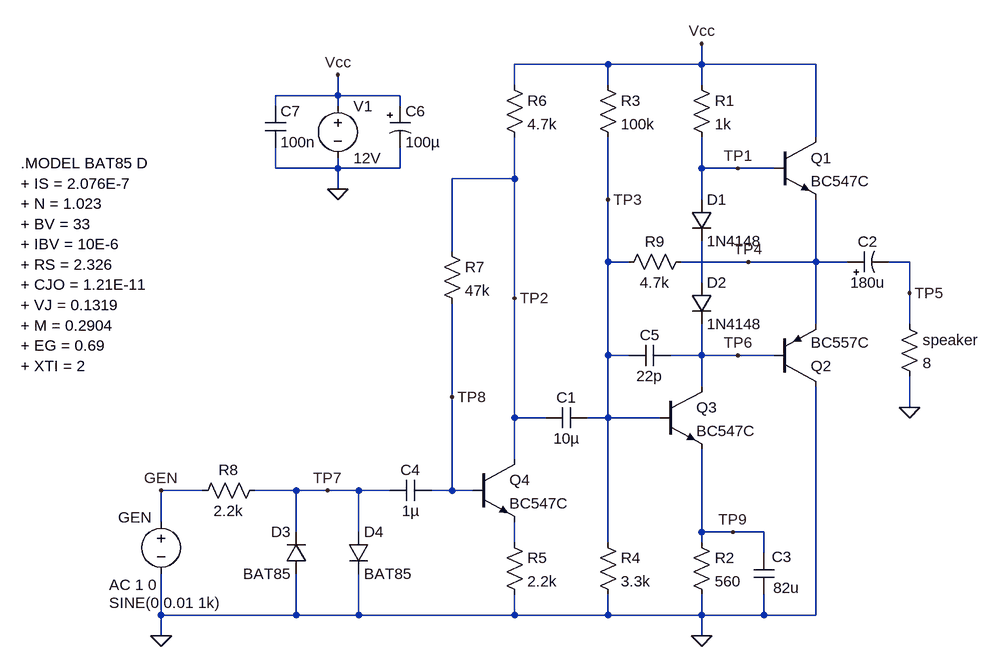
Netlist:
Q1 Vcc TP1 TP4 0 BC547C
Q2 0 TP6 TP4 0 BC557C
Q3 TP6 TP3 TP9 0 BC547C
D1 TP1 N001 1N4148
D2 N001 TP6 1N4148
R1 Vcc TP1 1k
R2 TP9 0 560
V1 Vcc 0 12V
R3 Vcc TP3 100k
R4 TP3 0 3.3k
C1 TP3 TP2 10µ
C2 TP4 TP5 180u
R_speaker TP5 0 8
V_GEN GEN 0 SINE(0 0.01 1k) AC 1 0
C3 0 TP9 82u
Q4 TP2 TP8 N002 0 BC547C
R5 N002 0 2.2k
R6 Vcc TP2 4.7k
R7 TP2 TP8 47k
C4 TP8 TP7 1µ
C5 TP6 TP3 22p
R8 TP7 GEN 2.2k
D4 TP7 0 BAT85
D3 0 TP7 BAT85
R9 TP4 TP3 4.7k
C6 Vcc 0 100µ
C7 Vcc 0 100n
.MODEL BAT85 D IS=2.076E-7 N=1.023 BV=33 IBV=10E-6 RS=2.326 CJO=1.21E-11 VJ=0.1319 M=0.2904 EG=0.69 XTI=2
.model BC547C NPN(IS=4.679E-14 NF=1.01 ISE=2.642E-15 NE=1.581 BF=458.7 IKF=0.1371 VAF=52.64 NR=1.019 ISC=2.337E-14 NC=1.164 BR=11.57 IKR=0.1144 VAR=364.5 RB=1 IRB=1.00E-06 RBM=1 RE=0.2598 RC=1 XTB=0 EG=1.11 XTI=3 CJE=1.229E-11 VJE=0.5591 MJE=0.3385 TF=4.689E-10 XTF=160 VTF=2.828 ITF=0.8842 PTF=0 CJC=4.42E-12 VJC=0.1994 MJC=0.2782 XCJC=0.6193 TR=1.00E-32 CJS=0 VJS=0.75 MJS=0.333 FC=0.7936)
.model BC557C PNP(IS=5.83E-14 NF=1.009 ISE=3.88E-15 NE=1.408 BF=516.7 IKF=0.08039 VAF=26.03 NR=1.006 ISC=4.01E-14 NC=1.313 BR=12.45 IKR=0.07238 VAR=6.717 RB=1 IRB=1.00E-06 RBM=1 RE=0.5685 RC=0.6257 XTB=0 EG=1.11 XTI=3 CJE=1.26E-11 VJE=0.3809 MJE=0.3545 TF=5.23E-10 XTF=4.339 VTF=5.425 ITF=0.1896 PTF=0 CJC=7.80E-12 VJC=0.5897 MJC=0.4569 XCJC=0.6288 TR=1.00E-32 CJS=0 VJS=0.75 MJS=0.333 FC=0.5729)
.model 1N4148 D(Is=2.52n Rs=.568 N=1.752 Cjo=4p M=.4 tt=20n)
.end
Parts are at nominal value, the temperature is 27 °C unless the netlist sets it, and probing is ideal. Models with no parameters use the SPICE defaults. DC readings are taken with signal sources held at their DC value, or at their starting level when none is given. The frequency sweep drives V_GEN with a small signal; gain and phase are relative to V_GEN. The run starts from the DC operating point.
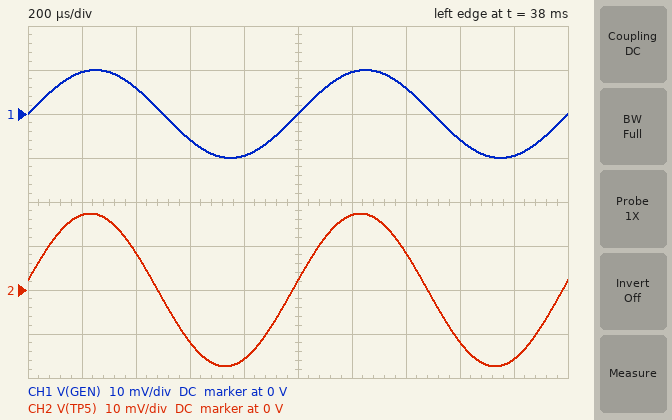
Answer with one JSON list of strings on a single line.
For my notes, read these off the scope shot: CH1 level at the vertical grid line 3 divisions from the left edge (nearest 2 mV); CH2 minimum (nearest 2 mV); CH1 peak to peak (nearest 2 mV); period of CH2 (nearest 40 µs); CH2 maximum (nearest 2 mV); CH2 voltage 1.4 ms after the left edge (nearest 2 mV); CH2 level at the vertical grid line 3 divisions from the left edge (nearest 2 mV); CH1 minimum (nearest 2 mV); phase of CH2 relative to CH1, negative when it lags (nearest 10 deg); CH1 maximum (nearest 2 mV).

["-6 mV", "-18 mV", "20 mV", "1.00 ms", "18 mV", "8 mV", "-12 mV", "-10 mV", "10 deg", "10 mV"]
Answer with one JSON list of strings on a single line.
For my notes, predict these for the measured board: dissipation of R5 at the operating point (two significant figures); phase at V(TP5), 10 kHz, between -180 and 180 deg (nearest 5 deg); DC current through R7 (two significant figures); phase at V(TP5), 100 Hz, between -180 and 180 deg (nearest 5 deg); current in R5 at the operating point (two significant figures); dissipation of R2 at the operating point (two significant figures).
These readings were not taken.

["5.8 mW", "0 deg", "3.6 µA", "55 deg", "1.6 mA", "10 mW"]
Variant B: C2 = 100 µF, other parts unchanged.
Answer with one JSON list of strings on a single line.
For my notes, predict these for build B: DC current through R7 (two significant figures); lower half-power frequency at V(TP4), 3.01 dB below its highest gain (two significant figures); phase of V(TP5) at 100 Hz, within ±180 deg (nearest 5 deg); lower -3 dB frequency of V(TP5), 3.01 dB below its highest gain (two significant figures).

["3.6 µA", "9.8 Hz", "70 deg", "200 Hz"]
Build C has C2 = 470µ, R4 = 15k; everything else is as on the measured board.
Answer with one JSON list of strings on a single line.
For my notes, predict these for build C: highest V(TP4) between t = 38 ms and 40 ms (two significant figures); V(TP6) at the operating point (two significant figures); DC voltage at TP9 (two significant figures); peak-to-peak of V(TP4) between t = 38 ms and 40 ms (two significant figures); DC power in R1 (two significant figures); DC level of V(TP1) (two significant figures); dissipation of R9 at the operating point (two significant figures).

["5.2 V", "4.5 V", "3.5 V", "36 mV", "38 mW", "5.8 V", "210 µW"]
